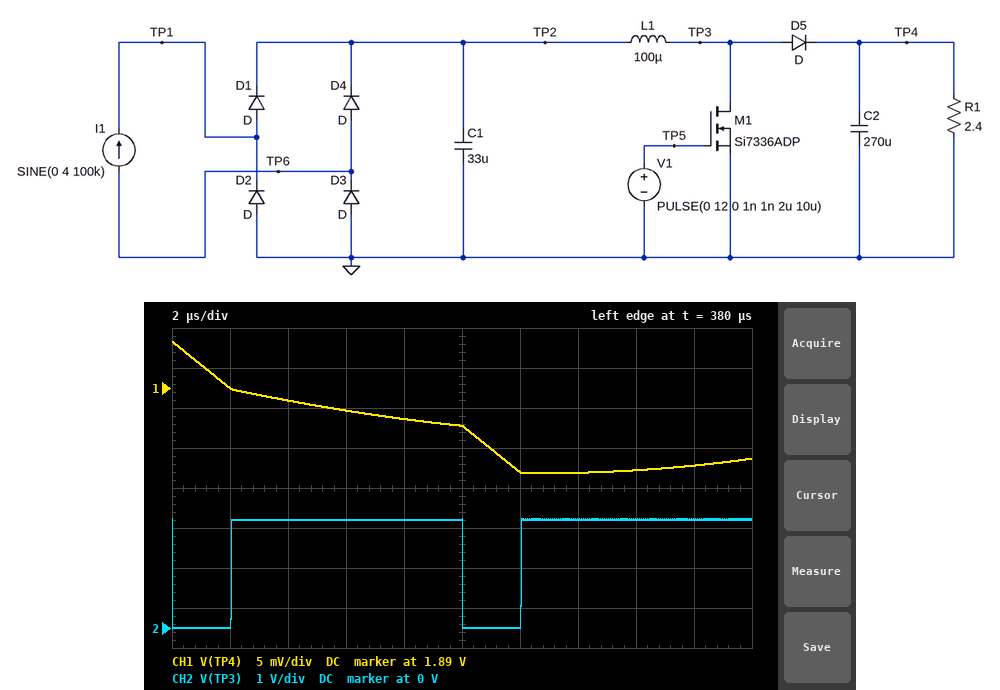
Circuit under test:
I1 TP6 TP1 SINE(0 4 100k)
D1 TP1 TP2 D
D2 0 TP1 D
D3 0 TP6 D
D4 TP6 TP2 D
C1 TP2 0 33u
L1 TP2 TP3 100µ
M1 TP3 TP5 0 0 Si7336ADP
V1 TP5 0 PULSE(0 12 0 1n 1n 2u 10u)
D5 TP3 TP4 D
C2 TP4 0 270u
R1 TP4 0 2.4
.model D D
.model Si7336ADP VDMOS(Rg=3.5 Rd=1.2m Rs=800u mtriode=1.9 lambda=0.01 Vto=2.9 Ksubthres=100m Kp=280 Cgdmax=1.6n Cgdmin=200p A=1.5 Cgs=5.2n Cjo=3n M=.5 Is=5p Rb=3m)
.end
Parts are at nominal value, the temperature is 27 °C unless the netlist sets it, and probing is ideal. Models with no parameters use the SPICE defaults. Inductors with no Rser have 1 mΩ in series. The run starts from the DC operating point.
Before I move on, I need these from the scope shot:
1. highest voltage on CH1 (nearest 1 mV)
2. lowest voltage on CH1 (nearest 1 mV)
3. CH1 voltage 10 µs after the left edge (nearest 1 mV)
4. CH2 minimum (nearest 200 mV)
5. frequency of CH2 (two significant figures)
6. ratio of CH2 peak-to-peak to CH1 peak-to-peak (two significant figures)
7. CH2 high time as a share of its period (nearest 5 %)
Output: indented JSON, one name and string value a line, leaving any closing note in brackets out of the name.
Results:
{
  "highest voltage on CH1": "1.896 V",
  "lowest voltage on CH1": "1.879 V",
  "CH1 voltage 10 µs after the left edge": "1.885 V",
  "CH2 minimum": "0 V",
  "frequency of CH2": "100 kHz",
  "ratio of CH2 peak-to-peak to CH1 peak-to-peak": "170",
  "CH2 high time as a share of its period": "80 %"
}
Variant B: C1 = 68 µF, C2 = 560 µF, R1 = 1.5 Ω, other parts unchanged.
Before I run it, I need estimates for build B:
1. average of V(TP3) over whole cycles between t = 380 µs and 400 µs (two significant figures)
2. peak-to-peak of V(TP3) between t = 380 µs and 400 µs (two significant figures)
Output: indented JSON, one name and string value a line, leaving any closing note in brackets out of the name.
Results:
{
  "average of V(TP3) over whole cycles between t = 380 µs and 400 µs": "1.7 V",
  "peak-to-peak of V(TP3) between t = 380 µs and 400 µs": "2.2 V"
}
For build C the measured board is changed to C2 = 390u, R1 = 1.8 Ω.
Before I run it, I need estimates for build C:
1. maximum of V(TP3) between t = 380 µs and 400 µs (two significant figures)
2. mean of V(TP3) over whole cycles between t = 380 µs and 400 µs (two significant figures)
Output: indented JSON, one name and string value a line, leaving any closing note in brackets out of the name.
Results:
{
  "maximum of V(TP3) between t = 380 µs and 400 µs": "2.3 V",
  "mean of V(TP3) over whole cycles between t = 380 µs and 400 µs": "1.8 V"
}
